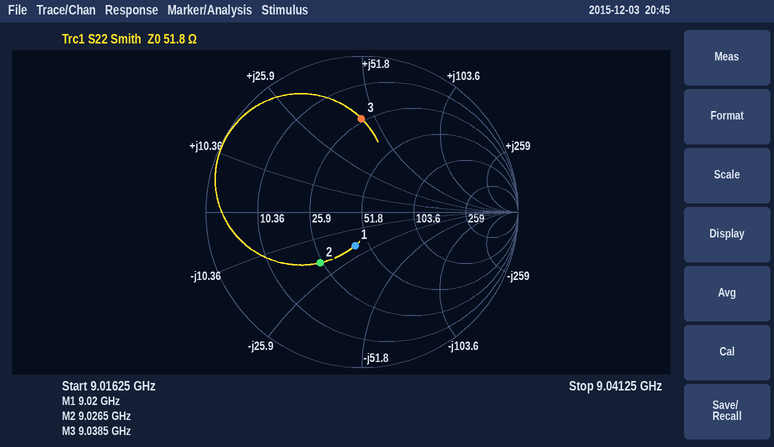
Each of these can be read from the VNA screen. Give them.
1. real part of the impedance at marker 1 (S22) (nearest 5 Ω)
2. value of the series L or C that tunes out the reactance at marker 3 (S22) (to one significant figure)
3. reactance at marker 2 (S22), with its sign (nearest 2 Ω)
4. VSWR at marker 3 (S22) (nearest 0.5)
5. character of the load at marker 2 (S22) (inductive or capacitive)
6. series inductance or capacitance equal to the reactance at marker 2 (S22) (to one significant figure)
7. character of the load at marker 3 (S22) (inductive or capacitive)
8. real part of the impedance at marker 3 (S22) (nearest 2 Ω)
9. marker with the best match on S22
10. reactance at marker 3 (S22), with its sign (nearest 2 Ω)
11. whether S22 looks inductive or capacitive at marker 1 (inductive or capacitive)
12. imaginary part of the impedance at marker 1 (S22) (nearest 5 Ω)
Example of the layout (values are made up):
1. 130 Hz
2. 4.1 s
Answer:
1. 45 Ω
2. 400 fF
3. -20 Ω
4. 4.0
5. capacitive
6. 900 fF
7. inductive
8. 24 Ω
9. marker 1
10. +46 Ω
11. capacitive
12. -20 Ω
